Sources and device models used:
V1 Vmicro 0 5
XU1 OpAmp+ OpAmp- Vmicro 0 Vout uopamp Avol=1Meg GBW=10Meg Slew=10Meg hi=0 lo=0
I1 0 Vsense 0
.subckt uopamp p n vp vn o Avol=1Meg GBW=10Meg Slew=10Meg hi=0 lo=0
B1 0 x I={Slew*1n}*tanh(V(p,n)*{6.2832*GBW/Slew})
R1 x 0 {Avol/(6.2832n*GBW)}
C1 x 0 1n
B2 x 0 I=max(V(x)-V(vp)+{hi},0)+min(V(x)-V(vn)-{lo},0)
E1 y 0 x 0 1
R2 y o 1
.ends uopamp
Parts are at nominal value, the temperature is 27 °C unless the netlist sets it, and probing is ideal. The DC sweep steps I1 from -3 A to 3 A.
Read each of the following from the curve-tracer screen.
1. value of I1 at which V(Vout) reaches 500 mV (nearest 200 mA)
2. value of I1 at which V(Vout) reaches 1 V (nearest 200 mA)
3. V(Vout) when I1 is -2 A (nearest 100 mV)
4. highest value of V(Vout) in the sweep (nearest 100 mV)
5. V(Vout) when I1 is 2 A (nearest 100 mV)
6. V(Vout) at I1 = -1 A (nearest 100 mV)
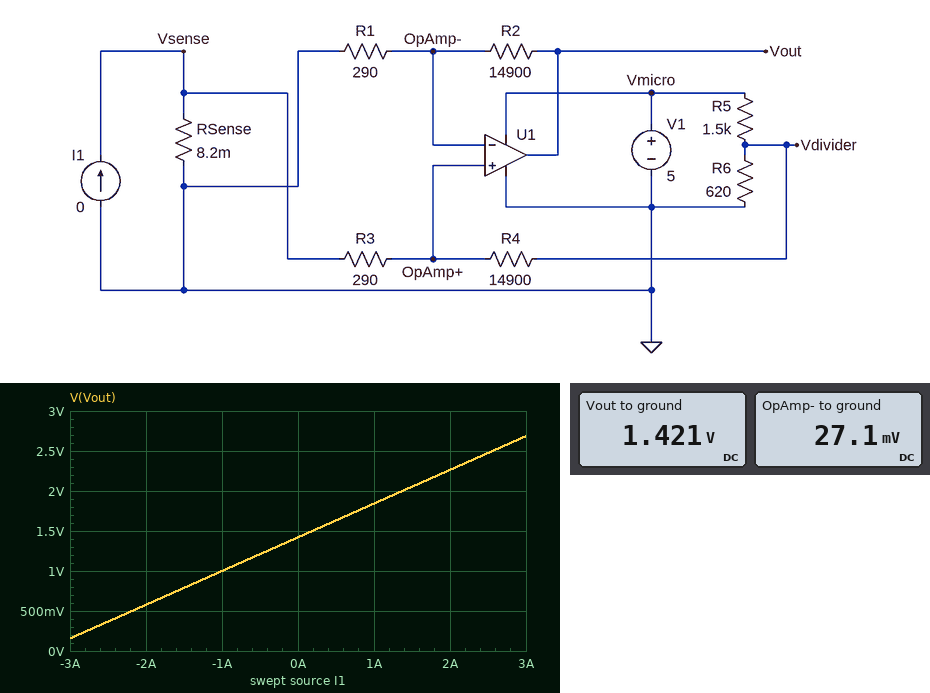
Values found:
-2.2 A
-1.0 A
600 mV
2.7 V
2.3 V
1.0 V
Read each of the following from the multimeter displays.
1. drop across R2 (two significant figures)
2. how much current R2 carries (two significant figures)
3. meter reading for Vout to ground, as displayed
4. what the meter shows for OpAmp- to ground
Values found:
1.4 V
94 µA
1.421 V
27.1 mV
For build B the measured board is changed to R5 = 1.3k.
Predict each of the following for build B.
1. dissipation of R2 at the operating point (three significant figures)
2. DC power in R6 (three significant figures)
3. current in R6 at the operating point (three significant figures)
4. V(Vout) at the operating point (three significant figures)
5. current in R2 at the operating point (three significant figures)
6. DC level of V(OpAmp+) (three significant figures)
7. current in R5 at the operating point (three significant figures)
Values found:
159 µW
3.98 mW
2.53 mA
1.57 V
103 µA
30.0 mV
2.64 mA
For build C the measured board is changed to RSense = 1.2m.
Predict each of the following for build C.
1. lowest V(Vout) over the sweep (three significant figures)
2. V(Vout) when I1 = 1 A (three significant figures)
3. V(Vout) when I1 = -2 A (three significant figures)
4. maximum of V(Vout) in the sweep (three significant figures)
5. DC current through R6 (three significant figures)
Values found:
1.24 V
1.48 V
1.30 V
1.61 V
2.29 mA
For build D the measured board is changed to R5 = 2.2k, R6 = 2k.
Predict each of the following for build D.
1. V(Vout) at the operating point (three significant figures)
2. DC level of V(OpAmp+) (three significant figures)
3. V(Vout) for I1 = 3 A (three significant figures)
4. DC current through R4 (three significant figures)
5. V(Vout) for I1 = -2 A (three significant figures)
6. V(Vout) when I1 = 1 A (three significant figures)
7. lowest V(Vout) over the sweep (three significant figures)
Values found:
2.23 V
42.5 mV
3.49 V
147 µA
1.38 V
2.65 V
962 mV
